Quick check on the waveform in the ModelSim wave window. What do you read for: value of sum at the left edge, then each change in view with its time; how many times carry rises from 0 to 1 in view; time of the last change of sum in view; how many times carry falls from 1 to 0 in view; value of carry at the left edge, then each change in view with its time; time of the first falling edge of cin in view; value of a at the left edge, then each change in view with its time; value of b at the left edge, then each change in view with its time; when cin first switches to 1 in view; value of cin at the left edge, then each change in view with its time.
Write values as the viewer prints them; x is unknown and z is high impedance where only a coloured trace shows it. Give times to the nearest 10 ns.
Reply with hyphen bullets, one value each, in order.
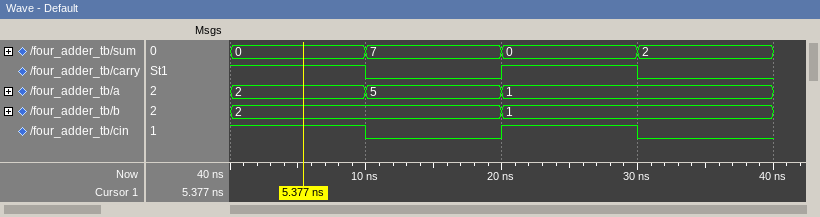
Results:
- 0, 7 at 10 ns, 0 at 20 ns, 2 at 30 ns
- 1
- 30 ns
- 2
- 1, 0 at 10 ns, 1 at 20 ns, 0 at 30 ns
- 10 ns
- 2, 5 at 10 ns, 1 at 20 ns
- 2, 1 at 20 ns
- 20 ns
- 1, 0 at 10 ns, 1 at 20 ns, 0 at 30 ns
